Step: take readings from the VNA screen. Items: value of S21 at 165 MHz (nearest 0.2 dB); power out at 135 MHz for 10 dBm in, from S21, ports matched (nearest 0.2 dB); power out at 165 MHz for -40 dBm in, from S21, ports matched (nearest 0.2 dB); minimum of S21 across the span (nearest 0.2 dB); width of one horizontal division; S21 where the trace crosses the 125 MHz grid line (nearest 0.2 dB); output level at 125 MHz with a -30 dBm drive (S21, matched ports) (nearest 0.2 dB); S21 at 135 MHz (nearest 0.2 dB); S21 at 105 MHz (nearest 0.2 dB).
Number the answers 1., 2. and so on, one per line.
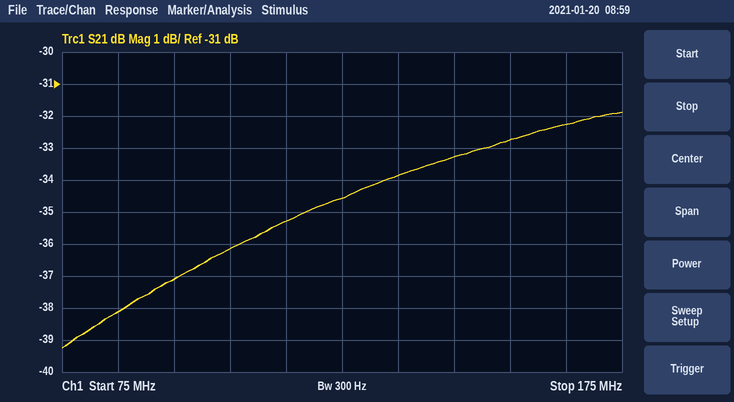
1. -32.2 dB
2. -23.8 dBm
3. -72.2 dBm
4. -39.2 dB
5. 10 MHz
6. -34.6 dB
7. -64.6 dBm
8. -33.8 dB
9. -36.2 dB
